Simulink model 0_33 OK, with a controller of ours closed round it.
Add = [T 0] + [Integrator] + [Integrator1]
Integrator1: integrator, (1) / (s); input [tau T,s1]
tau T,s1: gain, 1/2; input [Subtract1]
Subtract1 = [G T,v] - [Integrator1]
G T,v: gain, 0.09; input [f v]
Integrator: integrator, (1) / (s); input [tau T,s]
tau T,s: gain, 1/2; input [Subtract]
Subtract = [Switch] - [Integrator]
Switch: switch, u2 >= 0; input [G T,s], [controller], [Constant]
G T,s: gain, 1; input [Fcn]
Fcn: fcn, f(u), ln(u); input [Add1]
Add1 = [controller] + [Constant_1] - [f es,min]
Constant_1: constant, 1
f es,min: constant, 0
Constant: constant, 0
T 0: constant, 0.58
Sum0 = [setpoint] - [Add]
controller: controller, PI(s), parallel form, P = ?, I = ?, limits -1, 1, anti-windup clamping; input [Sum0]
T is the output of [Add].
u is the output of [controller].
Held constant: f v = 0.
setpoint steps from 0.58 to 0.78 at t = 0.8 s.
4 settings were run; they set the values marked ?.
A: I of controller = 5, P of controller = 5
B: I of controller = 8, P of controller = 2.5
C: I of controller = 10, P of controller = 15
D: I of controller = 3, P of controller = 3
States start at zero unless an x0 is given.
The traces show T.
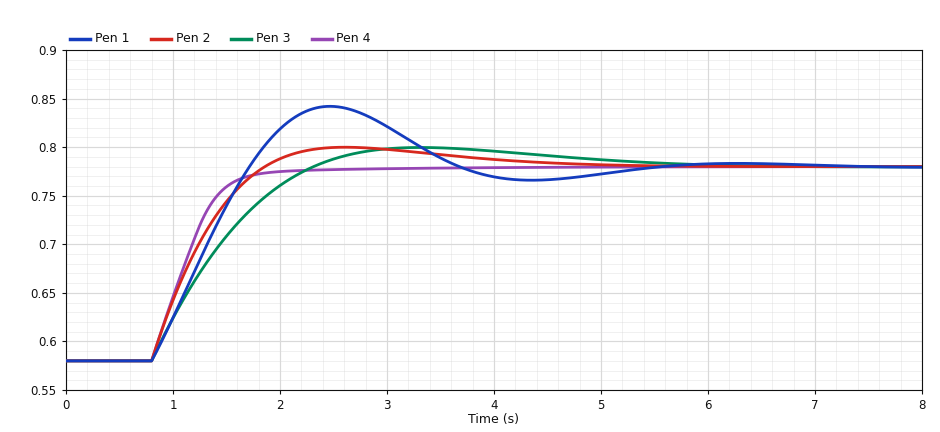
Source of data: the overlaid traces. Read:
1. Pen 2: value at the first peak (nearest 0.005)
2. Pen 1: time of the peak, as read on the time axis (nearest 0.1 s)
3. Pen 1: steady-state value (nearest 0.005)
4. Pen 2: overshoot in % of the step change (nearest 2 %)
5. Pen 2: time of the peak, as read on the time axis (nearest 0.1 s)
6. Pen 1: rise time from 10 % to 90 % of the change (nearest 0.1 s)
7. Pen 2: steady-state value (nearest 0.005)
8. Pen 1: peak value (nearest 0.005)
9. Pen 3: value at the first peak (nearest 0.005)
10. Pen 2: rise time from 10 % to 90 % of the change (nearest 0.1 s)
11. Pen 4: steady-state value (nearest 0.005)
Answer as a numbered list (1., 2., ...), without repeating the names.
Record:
1. 0.800
2. 2.5 s
3. 0.780
4. 10 %
5. 2.6 s
6. 0.7 s
7. 0.780
8. 0.840
9. 0.800
10. 0.8 s
11. 0.780
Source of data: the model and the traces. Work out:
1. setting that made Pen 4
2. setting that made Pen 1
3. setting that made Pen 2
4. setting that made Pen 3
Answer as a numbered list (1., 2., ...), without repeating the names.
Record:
1. C
2. B
3. A
4. D
